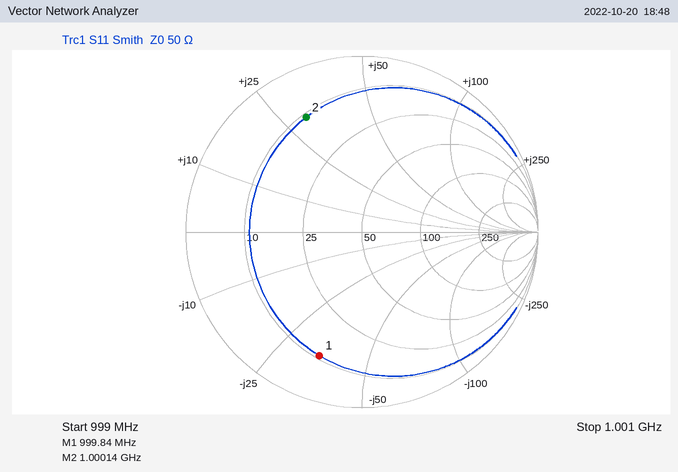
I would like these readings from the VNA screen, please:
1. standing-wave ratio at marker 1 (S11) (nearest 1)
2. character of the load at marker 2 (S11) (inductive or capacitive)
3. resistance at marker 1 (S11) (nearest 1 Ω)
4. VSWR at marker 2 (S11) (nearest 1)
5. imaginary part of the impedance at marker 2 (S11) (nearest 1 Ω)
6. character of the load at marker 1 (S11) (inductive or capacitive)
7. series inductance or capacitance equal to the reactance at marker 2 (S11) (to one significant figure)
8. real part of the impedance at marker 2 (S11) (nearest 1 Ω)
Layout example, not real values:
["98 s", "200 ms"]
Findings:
["7", "inductive", "11 Ω", "6", "+30 Ω", "capacitive", "5 nH", "11 Ω"]
